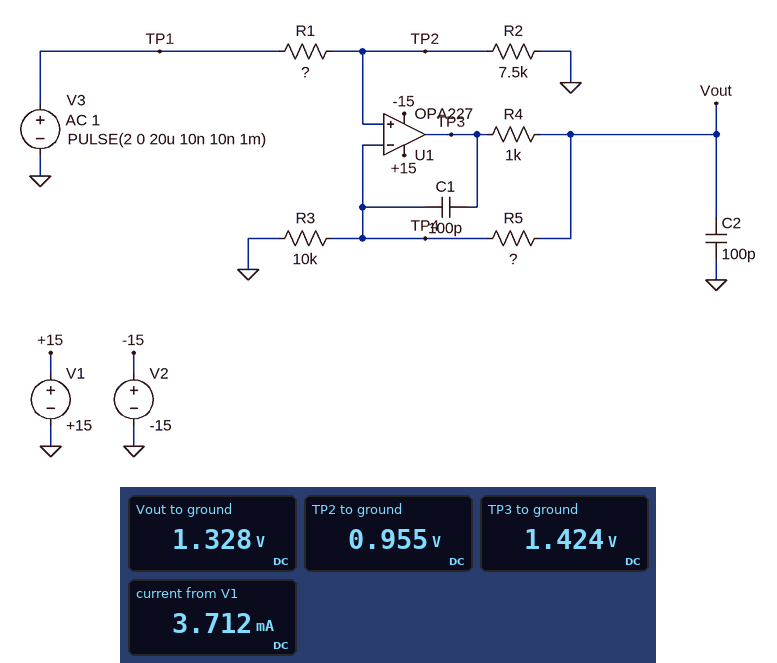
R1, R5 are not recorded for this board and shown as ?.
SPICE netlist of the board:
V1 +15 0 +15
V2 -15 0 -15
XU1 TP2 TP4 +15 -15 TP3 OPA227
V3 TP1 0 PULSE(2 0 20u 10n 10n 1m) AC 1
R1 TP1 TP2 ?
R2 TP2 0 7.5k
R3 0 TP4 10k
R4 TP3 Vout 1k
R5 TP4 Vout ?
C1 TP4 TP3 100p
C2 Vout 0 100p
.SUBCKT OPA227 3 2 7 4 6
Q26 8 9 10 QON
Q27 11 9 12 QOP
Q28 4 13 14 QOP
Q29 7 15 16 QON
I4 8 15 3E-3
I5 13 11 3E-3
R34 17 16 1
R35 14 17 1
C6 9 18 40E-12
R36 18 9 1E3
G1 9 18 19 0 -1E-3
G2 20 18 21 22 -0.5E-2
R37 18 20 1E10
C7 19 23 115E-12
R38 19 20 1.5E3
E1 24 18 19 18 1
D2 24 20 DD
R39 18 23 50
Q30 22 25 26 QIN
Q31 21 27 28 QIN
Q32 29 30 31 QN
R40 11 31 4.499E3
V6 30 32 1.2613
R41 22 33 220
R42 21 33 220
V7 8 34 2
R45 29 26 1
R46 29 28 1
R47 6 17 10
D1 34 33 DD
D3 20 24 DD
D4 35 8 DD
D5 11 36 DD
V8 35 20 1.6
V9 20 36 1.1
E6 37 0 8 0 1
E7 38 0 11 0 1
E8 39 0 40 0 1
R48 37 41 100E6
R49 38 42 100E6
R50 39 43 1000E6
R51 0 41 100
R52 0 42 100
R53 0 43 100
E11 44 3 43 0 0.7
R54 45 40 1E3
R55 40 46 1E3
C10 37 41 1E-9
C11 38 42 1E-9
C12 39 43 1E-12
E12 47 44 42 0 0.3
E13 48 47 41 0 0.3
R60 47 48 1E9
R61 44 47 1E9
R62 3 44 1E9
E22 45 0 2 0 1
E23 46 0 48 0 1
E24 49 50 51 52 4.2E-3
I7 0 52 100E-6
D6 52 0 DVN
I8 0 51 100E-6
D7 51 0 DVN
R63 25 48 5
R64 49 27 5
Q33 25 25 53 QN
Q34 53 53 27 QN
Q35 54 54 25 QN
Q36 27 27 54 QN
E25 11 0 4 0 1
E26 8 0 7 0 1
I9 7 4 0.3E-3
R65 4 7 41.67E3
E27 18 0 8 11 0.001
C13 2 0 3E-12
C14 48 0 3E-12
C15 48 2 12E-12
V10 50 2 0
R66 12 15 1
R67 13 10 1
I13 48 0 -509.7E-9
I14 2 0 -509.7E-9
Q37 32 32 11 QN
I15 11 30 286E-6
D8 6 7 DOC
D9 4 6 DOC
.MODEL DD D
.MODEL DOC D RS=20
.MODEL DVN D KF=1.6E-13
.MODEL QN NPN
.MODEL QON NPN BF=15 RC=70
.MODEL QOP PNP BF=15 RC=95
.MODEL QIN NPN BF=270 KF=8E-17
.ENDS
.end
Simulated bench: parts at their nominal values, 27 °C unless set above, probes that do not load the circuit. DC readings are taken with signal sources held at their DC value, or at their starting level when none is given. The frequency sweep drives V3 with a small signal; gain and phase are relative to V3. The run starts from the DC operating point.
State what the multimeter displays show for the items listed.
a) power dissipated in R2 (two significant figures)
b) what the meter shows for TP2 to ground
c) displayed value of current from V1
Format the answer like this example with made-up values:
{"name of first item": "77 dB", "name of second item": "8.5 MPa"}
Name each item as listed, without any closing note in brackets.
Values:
{"power dissipated in R2": "120 µW", "what the meter shows for TP2 to ground": "0.955 V", "displayed value of current from V1": "3.712 mA"}
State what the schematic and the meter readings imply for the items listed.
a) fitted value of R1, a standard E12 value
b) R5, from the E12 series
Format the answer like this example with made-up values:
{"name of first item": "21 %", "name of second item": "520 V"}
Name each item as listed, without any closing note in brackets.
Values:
{"fitted value of R1, a standard E12 value": "8.2 kΩ", "R5, from the E12 series": "3.9 kΩ"}
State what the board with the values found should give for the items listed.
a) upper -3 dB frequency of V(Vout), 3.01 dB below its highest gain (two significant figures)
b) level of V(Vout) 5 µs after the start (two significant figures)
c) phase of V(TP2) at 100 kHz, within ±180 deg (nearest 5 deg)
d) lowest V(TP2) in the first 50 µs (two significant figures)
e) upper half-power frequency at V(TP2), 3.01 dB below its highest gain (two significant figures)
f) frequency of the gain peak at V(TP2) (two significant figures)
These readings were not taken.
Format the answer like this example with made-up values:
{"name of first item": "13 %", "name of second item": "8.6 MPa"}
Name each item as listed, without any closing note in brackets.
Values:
{"upper -3 dB frequency of V(Vout), 3.01 dB below its highest gain": "3.6 MHz", "level of V(Vout) 5 µs after the start": "1.3 V", "phase of V(TP2) at 100 kHz, within ±180 deg": "0 deg", "lowest V(TP2) in the first 50 µs": "-76 mV", "upper half-power frequency at V(TP2), 3.01 dB below its highest gain": "4.2 MHz", "frequency of the gain peak at V(TP2)": "3.4 MHz"}
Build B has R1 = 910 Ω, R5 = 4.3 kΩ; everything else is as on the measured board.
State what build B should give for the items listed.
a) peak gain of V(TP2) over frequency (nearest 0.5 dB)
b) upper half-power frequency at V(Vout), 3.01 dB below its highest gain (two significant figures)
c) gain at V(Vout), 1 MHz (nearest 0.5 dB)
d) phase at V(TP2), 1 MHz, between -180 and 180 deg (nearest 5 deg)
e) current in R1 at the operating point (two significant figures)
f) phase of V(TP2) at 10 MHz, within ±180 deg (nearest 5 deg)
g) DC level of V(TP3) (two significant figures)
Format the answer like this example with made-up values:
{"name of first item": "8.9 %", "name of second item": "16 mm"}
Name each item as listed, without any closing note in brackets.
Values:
{"peak gain of V(TP2) over frequency": "1.0 dB", "upper half-power frequency at V(Vout), 3.01 dB below its highest gain": "1.3 MHz", "gain at V(Vout), 1 MHz": "0 dB", "phase at V(TP2), 1 MHz, between -180 and 180 deg": "0 deg", "current in R1 at the operating point": "240 µA", "phase of V(TP2) at 10 MHz, within ±180 deg": "-45 deg", "DC level of V(TP3)": "2.7 V"}
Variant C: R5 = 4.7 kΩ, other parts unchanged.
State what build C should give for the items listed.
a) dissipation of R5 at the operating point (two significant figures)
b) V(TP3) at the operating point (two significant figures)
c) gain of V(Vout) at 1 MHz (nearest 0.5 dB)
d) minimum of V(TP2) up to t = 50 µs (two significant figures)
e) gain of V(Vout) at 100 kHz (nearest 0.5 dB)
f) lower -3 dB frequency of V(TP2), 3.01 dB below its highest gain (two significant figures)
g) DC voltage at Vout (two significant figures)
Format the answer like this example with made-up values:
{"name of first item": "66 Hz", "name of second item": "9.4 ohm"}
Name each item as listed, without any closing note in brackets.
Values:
{"dissipation of R5 at the operating point": "43 µW", "V(TP3) at the operating point": "1.5 V", "gain of V(Vout) at 1 MHz": "-5.5 dB", "minimum of V(TP2) up to t = 50 µs": "-75 mV", "gain of V(Vout) at 100 kHz": "-3.0 dB", "lower -3 dB frequency of V(TP2), 3.01 dB below its highest gain": "2.2 MHz", "DC voltage at Vout": "1.4 V"}
